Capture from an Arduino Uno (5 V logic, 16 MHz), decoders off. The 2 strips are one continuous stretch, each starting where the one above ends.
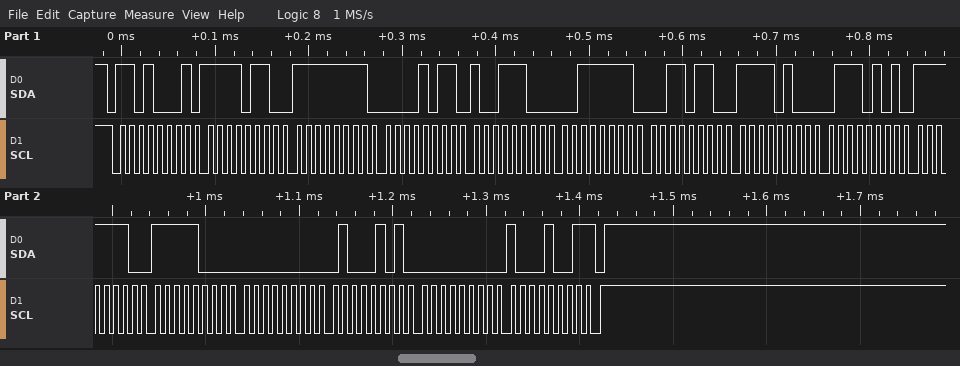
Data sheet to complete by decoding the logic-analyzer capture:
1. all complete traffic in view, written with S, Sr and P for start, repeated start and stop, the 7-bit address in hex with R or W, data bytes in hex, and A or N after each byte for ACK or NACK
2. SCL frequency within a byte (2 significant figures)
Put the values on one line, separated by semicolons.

S 68R A F6 A FF A 0B A 9C A 3F A 36 A F4 A 75 A FE A F8 A 00 A 45 A 00 A 89 N P; 100 kHz
